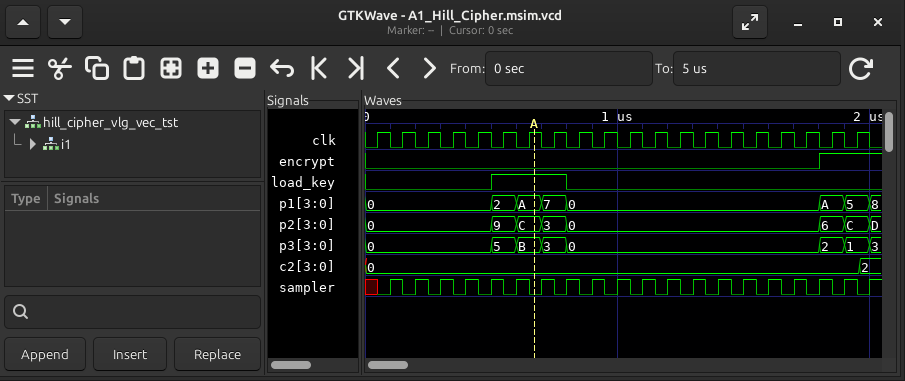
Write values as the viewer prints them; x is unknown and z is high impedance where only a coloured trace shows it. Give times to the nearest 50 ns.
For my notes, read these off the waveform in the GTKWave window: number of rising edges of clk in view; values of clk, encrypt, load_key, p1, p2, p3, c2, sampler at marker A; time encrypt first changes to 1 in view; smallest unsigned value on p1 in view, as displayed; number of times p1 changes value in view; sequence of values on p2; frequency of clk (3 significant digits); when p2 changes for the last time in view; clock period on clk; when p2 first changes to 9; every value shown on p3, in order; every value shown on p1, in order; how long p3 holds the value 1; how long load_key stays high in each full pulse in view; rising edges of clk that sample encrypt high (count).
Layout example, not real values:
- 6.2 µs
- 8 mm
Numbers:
- 20
- clk=1, encrypt=0, load_key=1, p1=A, p2=C, p3=B, c2=0, sampler=0
- 1800 ns
- 0
- 7
- 0, 9, C, 3, 0, 6, C, D
- 10.0 MHz
- 2000 ns
- 100 ns
- 500 ns
- 0, 5, B, 3, 0, 2, 1, 3
- 0, 2, A, 7, 0, A, 5, 8
- 100 ns
- 300 ns
- 2
